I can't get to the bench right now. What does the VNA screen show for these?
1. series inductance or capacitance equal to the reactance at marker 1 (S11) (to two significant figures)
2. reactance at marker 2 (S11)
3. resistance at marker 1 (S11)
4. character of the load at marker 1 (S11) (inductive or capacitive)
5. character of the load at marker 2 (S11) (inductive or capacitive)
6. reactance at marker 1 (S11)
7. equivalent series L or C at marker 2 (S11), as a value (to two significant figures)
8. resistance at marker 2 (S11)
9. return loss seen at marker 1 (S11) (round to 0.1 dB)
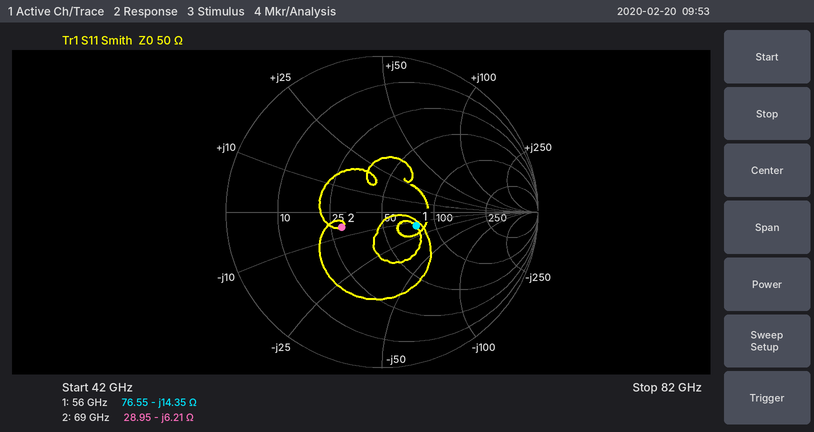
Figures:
200 fF
-6.21 Ω
76.55 Ω
capacitive
capacitive
-14.35 Ω
370 fF
28.95 Ω
12.5 dB
